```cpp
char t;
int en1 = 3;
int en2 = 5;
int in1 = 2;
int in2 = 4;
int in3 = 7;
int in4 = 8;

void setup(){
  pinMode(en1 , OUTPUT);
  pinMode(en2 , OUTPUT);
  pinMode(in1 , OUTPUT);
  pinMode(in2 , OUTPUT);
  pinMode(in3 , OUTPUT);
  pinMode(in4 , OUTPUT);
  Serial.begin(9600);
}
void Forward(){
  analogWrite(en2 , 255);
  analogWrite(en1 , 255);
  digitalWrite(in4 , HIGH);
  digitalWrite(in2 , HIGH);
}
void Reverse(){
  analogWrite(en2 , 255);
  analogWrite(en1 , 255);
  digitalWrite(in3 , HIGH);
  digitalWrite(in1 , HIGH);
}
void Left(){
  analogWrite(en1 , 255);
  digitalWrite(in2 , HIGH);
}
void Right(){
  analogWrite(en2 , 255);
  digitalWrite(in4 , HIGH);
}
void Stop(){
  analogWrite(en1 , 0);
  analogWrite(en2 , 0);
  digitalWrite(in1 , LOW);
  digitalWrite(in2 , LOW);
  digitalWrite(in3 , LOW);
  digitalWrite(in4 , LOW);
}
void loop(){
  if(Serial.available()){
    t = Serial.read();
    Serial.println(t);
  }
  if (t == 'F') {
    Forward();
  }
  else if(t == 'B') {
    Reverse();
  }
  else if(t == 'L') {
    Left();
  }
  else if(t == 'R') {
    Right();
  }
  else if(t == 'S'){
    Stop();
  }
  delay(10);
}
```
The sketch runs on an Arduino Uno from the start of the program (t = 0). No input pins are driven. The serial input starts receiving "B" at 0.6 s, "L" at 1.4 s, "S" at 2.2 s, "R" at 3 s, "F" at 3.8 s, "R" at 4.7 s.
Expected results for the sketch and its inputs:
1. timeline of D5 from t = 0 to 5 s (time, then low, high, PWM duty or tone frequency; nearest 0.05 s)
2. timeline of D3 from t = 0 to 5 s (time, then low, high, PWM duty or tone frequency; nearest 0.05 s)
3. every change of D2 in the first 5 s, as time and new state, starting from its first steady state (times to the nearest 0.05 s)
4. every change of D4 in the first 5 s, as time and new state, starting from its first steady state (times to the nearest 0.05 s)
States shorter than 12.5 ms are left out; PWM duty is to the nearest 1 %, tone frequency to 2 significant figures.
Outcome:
0 s low; 0.6 s high; 2.2 s low; 3 s high
0 s low; 0.6 s high; 2.2 s low; 3.8 s high
0 s low; 0.6 s high; 2.2 s low
0 s low; 1.4 s high; 2.2 s low; 3.8 s high
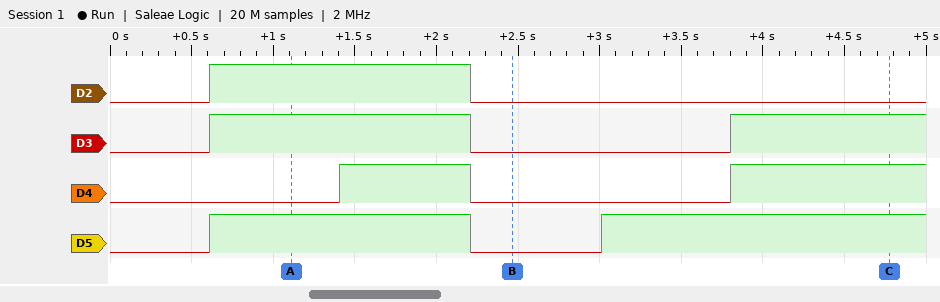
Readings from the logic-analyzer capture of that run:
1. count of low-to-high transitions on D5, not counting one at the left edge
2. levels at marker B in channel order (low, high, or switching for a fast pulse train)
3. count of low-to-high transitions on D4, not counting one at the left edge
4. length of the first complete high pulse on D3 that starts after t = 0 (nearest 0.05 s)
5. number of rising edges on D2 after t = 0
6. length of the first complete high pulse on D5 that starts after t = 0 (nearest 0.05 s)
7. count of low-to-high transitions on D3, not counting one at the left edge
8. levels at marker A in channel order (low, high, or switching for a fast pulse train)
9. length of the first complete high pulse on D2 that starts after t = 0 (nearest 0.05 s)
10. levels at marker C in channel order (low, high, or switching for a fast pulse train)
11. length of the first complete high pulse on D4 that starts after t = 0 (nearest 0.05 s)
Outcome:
2
D2 low, D3 low, D4 low, D5 low
2
1.60 s
1
1.60 s
2
D2 high, D3 high, D4 low, D5 high
1.60 s
D2 low, D3 high, D4 high, D5 high
0.80 s
